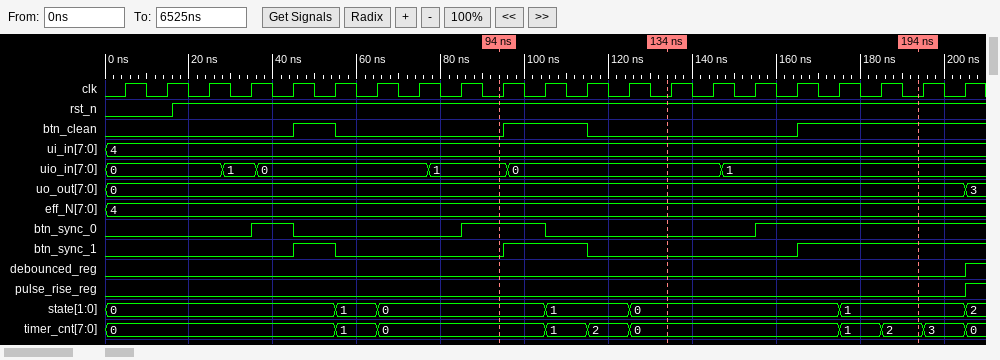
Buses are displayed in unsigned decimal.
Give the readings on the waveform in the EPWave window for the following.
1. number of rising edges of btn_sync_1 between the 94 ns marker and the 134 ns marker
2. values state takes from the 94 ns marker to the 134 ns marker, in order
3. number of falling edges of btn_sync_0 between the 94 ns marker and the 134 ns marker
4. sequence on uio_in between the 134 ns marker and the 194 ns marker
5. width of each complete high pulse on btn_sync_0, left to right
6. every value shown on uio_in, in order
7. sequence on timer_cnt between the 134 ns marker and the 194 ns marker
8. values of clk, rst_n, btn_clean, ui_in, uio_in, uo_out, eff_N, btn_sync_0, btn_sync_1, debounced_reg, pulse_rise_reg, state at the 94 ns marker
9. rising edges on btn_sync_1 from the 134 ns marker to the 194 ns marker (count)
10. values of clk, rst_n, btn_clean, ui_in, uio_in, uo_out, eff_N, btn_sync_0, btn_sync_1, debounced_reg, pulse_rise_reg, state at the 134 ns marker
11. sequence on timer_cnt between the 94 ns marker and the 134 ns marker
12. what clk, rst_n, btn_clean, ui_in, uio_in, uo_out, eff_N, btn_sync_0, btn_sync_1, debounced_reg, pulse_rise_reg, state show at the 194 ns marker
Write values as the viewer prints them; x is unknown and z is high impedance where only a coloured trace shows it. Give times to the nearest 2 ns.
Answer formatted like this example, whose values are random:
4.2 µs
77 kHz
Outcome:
1
0, 1, 0
1
0, 1
10 ns, 20 ns
0, 1, 0, 1, 0, 1
0, 1, 2
clk=0, rst_n=1, btn_clean=0, ui_in=4, uio_in=1, uo_out=0, eff_N=4, btn_sync_0=1, btn_sync_1=0, debounced_reg=0, pulse_rise_reg=0, state=0
1
clk=0, rst_n=1, btn_clean=0, ui_in=4, uio_in=0, uo_out=0, eff_N=4, btn_sync_0=0, btn_sync_1=0, debounced_reg=0, pulse_rise_reg=0, state=0
0, 1, 2, 0
clk=0, rst_n=1, btn_clean=1, ui_in=4, uio_in=1, uo_out=0, eff_N=4, btn_sync_0=1, btn_sync_1=1, debounced_reg=0, pulse_rise_reg=0, state=1
